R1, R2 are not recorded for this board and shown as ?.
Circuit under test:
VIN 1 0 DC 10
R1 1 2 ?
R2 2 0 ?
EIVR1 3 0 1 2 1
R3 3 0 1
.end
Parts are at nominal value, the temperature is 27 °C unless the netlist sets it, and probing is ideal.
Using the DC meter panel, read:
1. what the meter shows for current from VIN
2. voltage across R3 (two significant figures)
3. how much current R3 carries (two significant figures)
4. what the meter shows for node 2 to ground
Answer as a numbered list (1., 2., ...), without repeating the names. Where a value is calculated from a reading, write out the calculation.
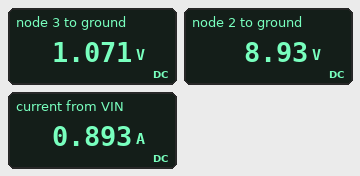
1. 0.893 A
2. 1.071 V = 1.1 V
3. (1.071 V) / 1 Ω = 1.1 A
4. 8.93 V
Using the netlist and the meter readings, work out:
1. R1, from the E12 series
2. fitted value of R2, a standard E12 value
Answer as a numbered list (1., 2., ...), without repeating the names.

1. 1.2 Ω
2. 10 Ω
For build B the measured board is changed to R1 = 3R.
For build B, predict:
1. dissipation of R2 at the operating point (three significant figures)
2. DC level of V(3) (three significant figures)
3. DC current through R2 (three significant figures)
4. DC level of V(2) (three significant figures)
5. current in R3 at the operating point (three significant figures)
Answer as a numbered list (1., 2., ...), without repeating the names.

1. 5.92 W
2. 2.31 V
3. 769 mA
4. 7.69 V
5. 2.31 A
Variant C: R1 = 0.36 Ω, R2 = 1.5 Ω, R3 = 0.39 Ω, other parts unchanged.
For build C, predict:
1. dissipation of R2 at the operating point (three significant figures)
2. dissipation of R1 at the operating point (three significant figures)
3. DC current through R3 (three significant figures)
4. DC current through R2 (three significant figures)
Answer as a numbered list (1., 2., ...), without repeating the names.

1. 43.4 W
2. 10.4 W
3. 4.96 A
4. 5.38 A
